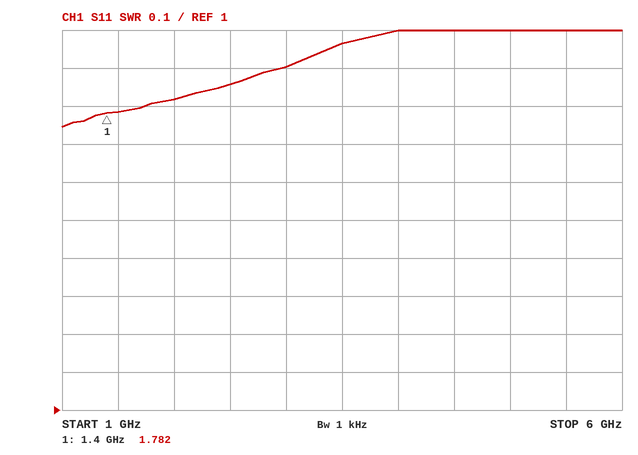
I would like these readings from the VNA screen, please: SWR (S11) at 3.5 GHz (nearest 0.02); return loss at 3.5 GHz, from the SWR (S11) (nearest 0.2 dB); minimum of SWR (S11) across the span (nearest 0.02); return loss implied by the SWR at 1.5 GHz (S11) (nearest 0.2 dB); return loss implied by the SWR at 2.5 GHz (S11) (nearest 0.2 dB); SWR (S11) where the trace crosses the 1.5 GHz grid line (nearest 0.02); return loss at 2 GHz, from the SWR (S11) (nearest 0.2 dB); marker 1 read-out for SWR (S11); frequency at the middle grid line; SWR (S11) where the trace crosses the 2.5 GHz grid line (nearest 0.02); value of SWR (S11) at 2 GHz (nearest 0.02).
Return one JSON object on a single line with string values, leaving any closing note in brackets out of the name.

{"SWR (S11) at 3.5 GHz": "1.96", "return loss at 3.5 GHz, from the SWR (S11)": "9.8 dB", "minimum of SWR (S11) across the span": "1.74", "return loss implied by the SWR at 1.5 GHz (S11)": "11.0 dB", "return loss implied by the SWR at 2.5 GHz (S11)": "10.4 dB", "SWR (S11) where the trace crosses the 1.5 GHz grid line": "1.78", "return loss at 2 GHz, from the SWR (S11)": "10.8 dB", "marker 1 read-out for SWR": "1.782", "frequency at the middle grid line": "3.5 GHz", "SWR (S11) where the trace crosses the 2.5 GHz grid line": "1.86", "value of SWR (S11) at 2 GHz": "1.82"}
